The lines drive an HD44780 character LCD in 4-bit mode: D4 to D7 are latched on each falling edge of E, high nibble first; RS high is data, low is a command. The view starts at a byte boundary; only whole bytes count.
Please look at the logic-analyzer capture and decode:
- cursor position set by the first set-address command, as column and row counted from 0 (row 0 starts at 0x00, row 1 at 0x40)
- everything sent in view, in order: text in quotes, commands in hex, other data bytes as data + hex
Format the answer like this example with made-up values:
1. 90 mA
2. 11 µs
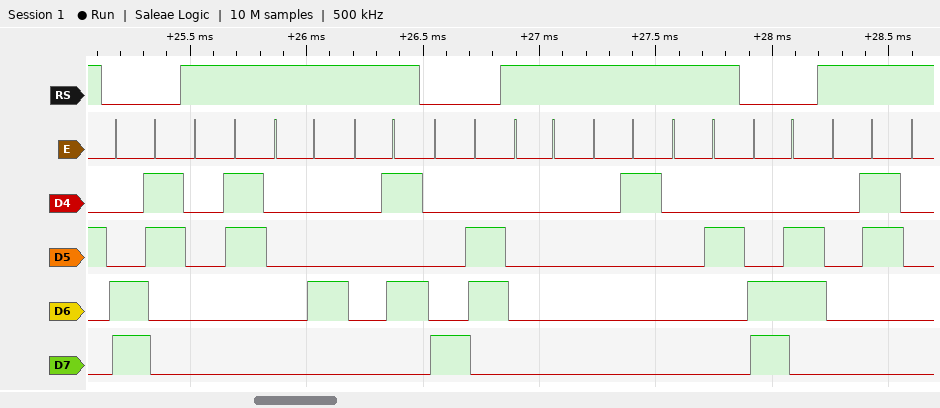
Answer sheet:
1. column 3, row 1
2. 0xC3 data 03 04 05 0x86 data 00 01 02 0xC6 data 03
